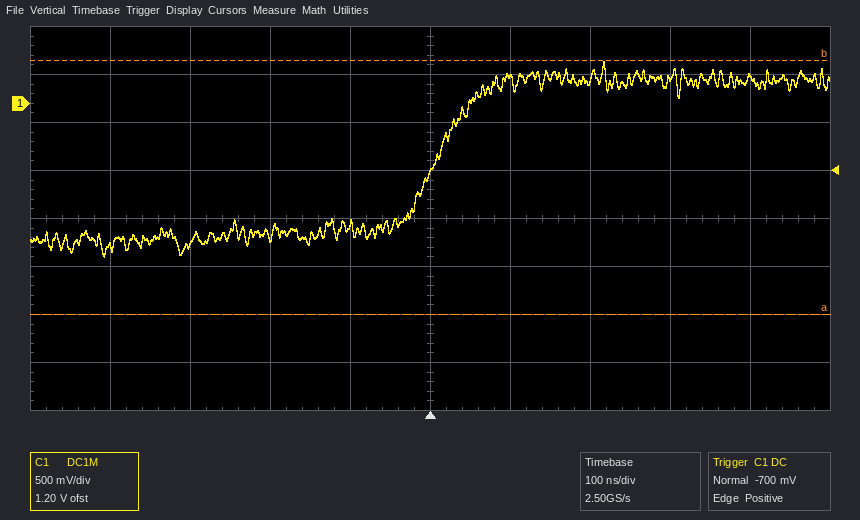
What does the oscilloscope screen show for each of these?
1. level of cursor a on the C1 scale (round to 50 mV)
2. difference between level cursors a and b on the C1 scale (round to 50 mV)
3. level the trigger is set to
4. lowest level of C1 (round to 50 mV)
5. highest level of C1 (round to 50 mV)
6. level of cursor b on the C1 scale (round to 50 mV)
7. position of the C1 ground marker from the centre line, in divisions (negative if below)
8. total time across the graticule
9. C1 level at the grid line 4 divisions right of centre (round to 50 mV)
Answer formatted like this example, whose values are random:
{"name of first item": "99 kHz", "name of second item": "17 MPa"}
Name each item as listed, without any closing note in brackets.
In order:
{"level of cursor a on the C1 scale": "-2.20 V", "difference between level cursors a and b on the C1 scale": "2.65 V", "level the trigger is set to": "-700 mV", "lowest level of C1": "-1.60 V", "highest level of C1": "450 mV", "level of cursor b on the C1 scale": "450 mV", "position of the C1 ground marker from the centre line, in divisions": "+2.4 div", "total time across the graticule": "1 µs", "C1 level at the grid line 4 divisions right of centre": "250 mV"}
